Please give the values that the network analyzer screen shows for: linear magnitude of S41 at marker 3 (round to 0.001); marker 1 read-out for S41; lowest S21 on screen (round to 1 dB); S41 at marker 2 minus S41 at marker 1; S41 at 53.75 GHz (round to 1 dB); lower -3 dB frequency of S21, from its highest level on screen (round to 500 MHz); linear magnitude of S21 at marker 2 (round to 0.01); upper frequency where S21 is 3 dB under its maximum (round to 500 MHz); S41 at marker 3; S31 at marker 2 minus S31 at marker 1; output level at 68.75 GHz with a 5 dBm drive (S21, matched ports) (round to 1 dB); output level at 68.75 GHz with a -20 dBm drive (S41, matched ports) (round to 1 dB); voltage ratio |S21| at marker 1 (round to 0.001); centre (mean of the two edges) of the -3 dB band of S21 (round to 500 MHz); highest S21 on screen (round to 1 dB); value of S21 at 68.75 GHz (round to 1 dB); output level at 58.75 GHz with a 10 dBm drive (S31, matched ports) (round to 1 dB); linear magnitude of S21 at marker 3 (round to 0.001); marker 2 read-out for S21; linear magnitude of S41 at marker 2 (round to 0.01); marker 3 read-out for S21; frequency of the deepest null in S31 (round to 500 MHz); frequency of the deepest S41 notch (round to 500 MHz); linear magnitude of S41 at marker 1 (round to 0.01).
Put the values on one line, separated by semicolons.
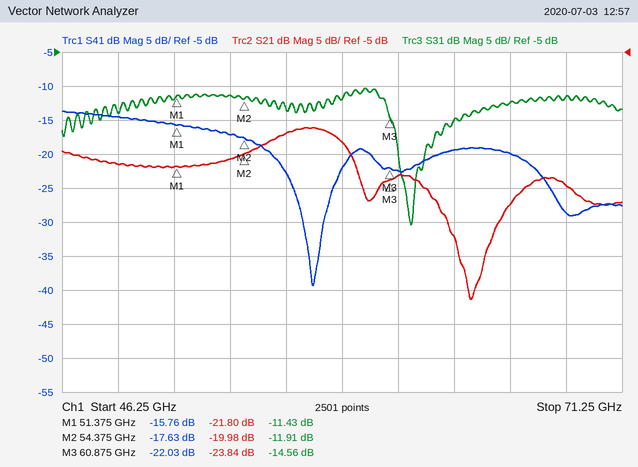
0.079; -15.76 dB; -41 dB; -1.87 dB; -17 dB; 55.0 GHz; 0.10; 59.0 GHz; -22.03 dB; -0.48 dB; -20 dBm; -49 dBm; 0.081; 57.0 GHz; -16 dB; -25 dB; -2 dBm; 0.064; -19.98 dB; 0.13; -23.84 dB; 62.0 GHz; 57.5 GHz; 0.16
